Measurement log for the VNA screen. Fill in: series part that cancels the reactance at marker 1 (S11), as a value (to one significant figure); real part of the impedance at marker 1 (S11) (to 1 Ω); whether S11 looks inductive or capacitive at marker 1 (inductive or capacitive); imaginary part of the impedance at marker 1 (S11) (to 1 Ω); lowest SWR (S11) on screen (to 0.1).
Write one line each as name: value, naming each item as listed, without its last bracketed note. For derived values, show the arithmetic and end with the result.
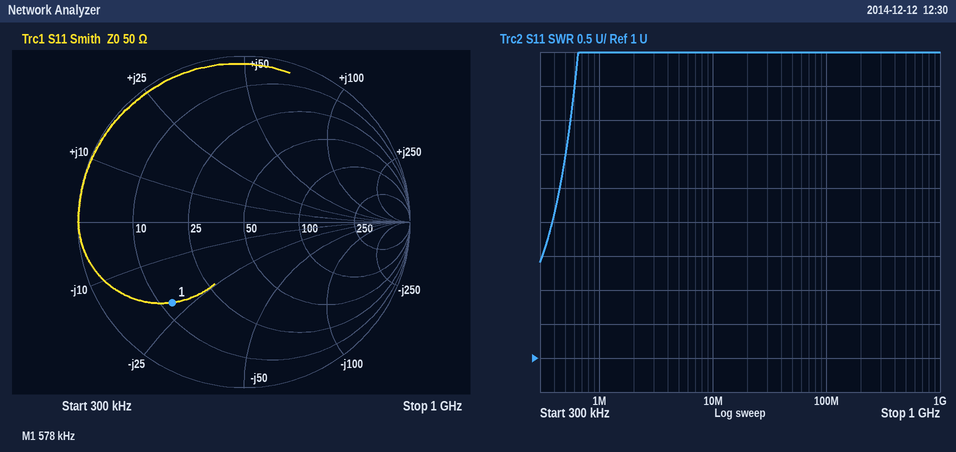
series part that cancels the reactance at marker 1 (S11), as a value: L = 21 Ω/(2π × 578 kHz) ≈ 6 µH
real part of the impedance at marker 1 (S11): 13 Ω
whether S11 looks inductive or capacitive at marker 1: capacitive
imaginary part of the impedance at marker 1 (S11): -21 Ω
lowest SWR (S11) on screen: 2.4
